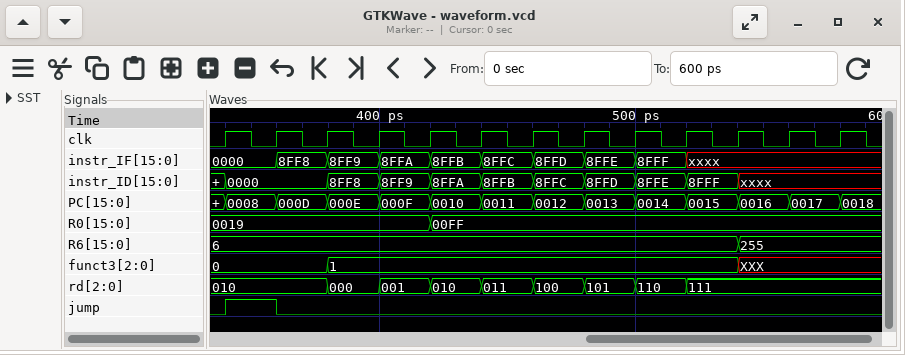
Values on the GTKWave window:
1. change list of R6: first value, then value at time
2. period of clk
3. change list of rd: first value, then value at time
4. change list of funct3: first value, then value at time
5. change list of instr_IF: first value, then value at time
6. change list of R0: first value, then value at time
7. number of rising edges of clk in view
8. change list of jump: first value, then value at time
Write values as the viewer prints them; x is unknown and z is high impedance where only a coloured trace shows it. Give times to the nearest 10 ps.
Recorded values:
6, 255 at 540 ps
20 ps
010, 000 at 380 ps, 001 at 400 ps, 010 at 420 ps, 011 at 440 ps, 100 at 460 ps, 101 at 480 ps, 110 at 500 ps, 111 at 520 ps
0, 1 at 380 ps, XXX at 540 ps
0000, 8FF8 at 360 ps, 8FF9 at 380 ps, 8FFA at 400 ps, 8FFB at 420 ps, 8FFC at 440 ps, 8FFD at 460 ps, 8FFE at 480 ps, 8FFF at 500 ps, xxxx at 520 ps
0019, 00FF at 420 ps
13
0, 1 at 340 ps, 0 at 360 ps
